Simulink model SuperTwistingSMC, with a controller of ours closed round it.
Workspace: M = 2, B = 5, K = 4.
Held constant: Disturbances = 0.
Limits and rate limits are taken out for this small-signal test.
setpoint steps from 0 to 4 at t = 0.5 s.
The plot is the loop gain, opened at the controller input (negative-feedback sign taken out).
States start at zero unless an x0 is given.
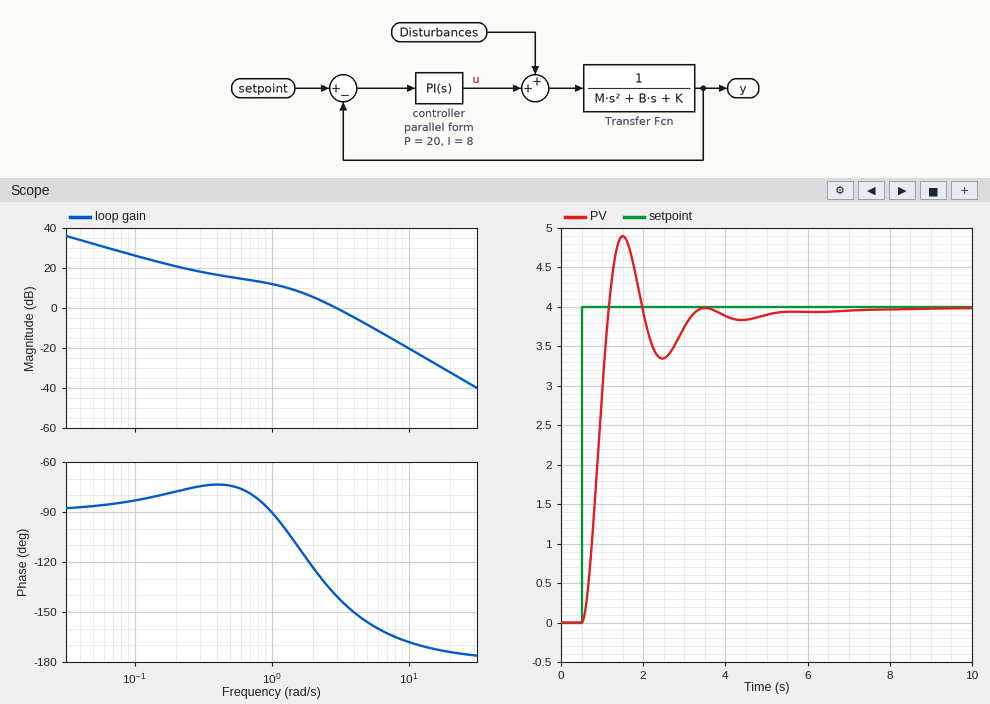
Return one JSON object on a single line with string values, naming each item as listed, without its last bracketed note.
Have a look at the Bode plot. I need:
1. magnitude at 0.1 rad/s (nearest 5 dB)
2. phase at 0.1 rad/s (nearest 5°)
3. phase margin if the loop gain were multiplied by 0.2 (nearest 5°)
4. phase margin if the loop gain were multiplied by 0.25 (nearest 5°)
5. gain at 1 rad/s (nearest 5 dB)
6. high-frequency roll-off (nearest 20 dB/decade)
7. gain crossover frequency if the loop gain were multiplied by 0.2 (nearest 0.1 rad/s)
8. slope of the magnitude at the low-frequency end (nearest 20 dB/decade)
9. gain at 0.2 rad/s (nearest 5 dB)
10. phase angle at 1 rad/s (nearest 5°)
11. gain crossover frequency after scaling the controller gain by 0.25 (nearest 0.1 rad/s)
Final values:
{"magnitude at 0.1 rad/s": "25 dB", "phase at 0.1 rad/s": "-85°", "phase margin if the loop gain were multiplied by 0.2": "100°", "phase margin if the loop gain were multiplied by 0.25": "90°", "gain at 1 rad/s": "10 dB", "high-frequency roll-off": "-40 dB/decade", "gain crossover frequency if the loop gain were multiplied by 0.2": "0.7 rad/s", "slope of the magnitude at the low-frequency end": "-20 dB/decade", "gain at 0.2 rad/s": "20 dB", "phase angle at 1 rad/s": "-90°", "gain crossover frequency after scaling the controller gain by 0.25": "1.0 rad/s"}
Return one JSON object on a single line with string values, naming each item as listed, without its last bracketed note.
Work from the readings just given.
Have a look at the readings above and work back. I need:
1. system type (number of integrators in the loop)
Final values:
{"system type": "1"}
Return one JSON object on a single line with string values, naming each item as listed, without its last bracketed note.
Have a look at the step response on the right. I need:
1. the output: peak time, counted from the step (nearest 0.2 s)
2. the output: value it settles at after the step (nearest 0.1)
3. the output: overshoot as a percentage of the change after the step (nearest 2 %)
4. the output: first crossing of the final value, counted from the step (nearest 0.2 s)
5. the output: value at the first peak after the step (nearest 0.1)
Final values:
{"the output: peak time, counted from the step": "1.0 s", "the output: value it settles at after the step": "4.0", "the output: overshoot as a percentage of the change after the step": "22 %", "the output: first crossing of the final value, counted from the step": "0.6 s", "the output: value at the first peak after the step": "4.9"}
